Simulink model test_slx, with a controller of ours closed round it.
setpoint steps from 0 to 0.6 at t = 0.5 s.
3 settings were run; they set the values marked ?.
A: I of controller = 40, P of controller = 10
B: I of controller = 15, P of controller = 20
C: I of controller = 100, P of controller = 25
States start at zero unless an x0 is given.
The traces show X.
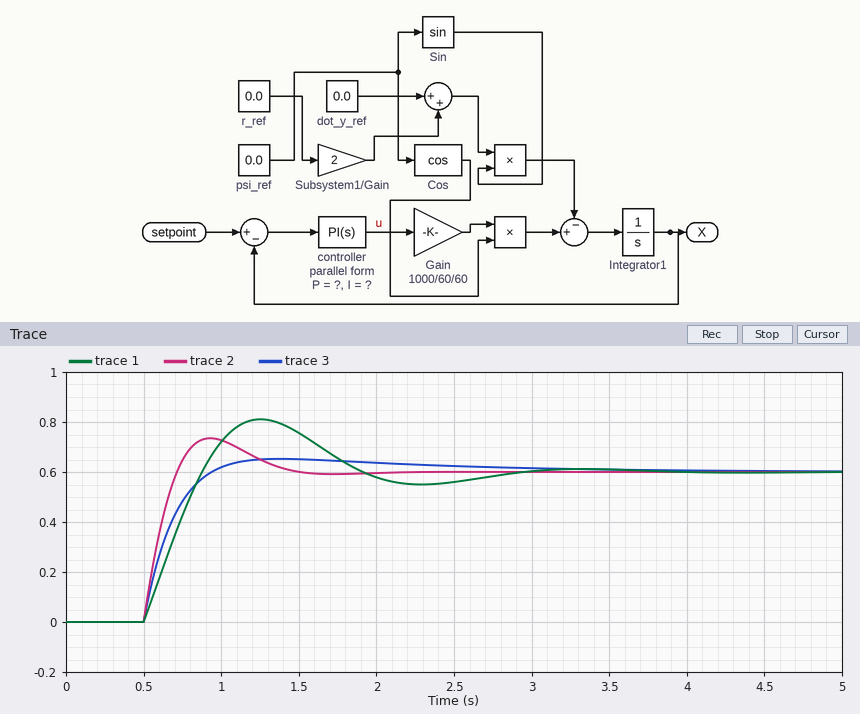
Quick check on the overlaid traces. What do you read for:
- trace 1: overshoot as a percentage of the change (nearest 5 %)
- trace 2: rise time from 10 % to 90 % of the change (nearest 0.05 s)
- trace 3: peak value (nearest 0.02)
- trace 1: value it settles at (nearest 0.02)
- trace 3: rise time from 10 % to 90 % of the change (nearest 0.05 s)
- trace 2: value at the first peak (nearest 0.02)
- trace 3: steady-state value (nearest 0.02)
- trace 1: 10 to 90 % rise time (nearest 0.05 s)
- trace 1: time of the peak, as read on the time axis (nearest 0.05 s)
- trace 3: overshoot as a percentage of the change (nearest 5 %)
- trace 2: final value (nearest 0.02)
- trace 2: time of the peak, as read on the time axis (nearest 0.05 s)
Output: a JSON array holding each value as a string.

["35 %", "0.15 s", "0.66", "0.60", "0.30 s", "0.74", "0.60", "0.30 s", "1.25 s", "10 %", "0.60", "0.95 s"]
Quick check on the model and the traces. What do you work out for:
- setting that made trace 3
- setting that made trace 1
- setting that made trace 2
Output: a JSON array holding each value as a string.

["B", "A", "C"]
